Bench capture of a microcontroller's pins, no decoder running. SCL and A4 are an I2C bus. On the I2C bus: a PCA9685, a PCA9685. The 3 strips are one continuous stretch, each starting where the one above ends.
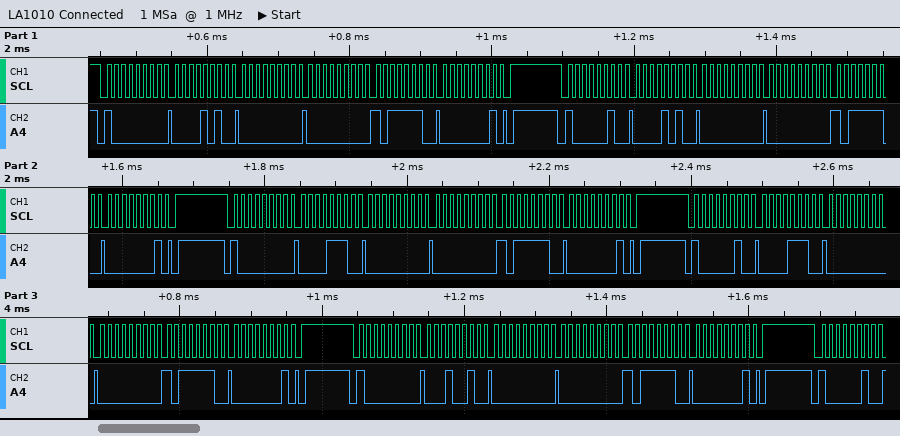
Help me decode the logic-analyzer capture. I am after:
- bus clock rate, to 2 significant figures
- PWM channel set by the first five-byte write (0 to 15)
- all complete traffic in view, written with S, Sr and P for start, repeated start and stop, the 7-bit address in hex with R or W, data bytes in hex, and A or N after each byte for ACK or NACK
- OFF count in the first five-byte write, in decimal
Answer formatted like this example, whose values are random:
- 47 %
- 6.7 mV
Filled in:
- 100 kHz
- 1
- S 40W A 0A A 00 A 00 A BE A 01 A P S 41W A 0A A 00 A 00 A BE A 01 A P S 40W A 0E A 00 A 00 A BE A 01 A P S 41W A 0E A 00 A 00 A BE A 01 A P S 40W A 12 A 00 A 00 A BE A 01 A P S 41W A
- 446
